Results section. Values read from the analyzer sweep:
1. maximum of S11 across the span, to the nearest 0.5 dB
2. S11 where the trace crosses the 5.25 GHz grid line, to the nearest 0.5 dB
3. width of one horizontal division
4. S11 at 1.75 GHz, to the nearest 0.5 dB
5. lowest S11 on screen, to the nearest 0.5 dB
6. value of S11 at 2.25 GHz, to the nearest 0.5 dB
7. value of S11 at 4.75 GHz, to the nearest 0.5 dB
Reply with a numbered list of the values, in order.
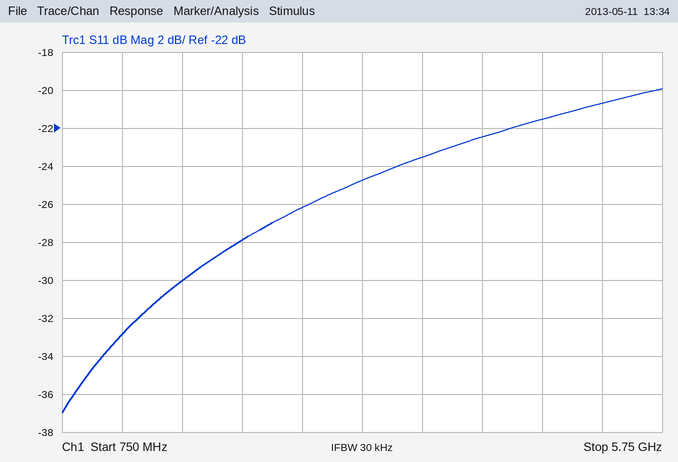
1. -20.0 dB
2. -20.5 dB
3. 500 MHz
4. -30.0 dB
5. -37.0 dB
6. -28.0 dB
7. -21.5 dB
